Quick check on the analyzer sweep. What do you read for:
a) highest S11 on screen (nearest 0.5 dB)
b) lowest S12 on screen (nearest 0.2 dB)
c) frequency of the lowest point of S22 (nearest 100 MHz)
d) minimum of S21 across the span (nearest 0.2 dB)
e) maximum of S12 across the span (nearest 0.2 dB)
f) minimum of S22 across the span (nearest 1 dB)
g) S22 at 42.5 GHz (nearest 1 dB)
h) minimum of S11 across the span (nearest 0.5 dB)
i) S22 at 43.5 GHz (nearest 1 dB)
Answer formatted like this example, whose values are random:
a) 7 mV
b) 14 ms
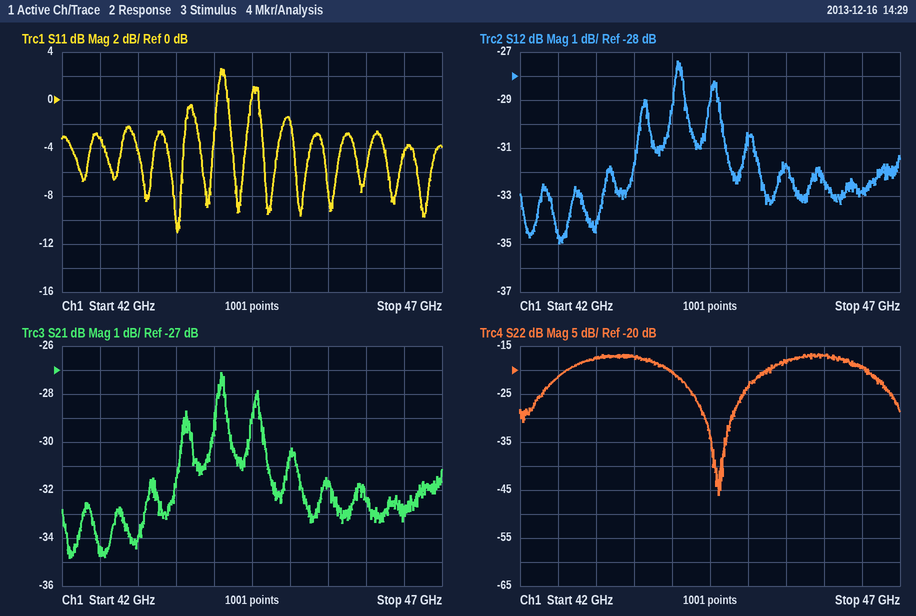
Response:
a) 2.5 dB
b) -35.0 dB
c) 44.6 GHz
d) -34.8 dB
e) -27.4 dB
f) -46 dB
g) -21 dB
h) -11.0 dB
i) -17 dB
